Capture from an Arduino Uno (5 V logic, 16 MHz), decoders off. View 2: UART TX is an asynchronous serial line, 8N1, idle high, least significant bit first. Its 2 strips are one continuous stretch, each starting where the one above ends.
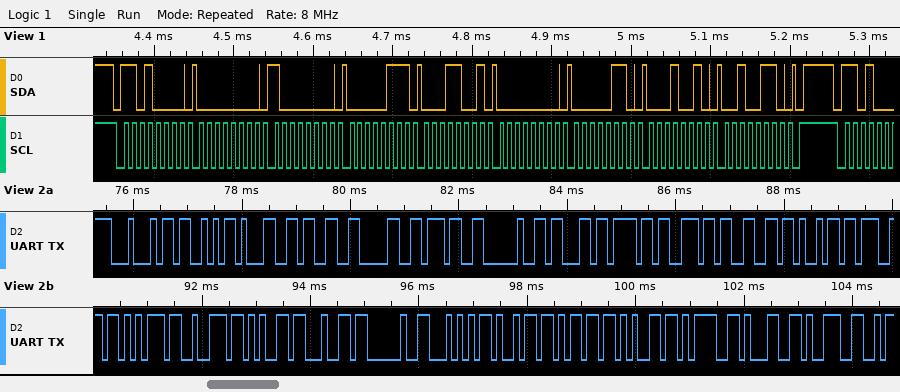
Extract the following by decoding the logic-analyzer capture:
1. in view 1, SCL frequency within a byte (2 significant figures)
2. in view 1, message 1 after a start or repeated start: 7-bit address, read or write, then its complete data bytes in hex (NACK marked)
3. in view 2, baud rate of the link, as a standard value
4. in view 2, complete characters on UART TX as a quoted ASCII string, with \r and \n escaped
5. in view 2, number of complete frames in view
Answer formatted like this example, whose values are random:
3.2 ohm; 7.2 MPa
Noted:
100 kHz; 0x68 write: 00 80 07 19 00 06 12 26; 9600 baud; "DS1307 configured Time=19"; 25
